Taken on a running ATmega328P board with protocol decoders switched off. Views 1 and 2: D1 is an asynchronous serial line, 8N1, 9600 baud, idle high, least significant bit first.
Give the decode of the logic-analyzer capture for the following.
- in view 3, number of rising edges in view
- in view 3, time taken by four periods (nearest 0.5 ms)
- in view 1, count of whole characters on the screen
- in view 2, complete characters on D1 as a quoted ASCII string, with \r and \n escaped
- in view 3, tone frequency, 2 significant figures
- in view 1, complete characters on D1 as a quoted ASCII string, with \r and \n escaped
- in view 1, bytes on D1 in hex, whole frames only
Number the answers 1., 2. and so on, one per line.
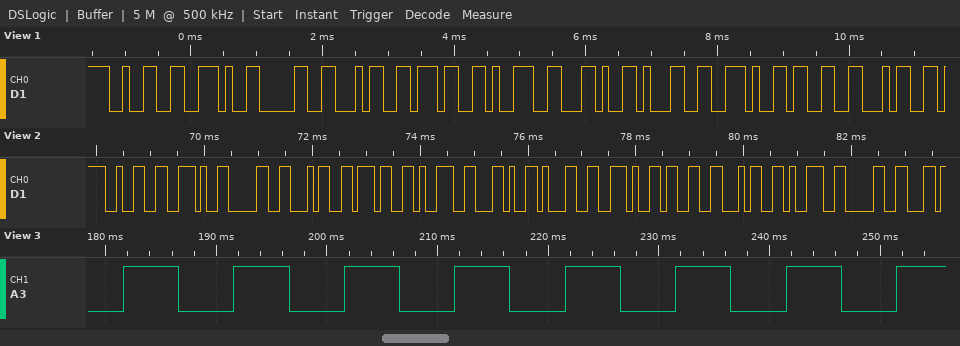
1. 8
2. 40.0 ms
3. 11
4. "2.0479,1.3490"
5. 100 Hz
6. "2.0479,1.34"
7. 32 2E 30 34 37 39 2C 31 2E 33 34
